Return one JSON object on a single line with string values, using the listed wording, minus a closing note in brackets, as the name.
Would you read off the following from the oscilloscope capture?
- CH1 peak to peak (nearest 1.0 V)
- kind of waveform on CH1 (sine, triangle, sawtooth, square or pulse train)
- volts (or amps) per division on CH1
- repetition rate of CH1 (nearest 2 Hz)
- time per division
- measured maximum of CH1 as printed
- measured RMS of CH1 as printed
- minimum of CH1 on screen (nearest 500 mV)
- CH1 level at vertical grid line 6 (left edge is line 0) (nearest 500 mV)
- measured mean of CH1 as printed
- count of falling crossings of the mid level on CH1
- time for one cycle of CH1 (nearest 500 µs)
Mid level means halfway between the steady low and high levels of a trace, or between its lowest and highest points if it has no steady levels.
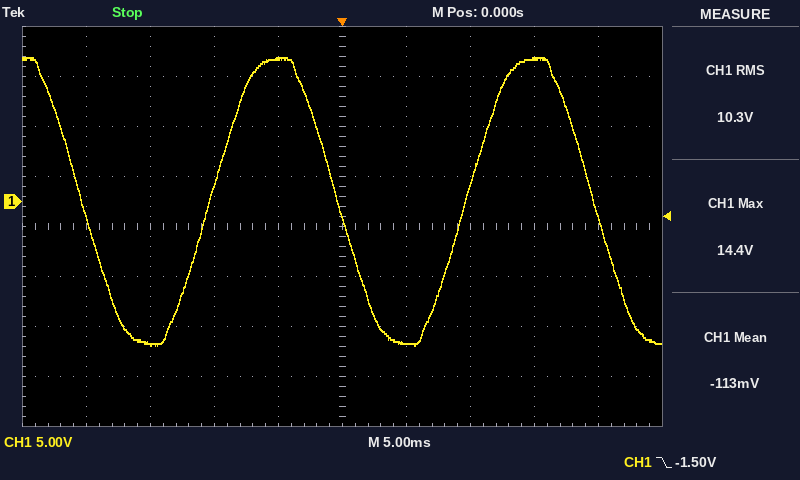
{"CH1 peak to peak": "29.0 V", "kind of waveform on CH1": "sine", "volts (or amps) per division on CH1": "5 V", "repetition rate of CH1": "50 Hz", "time per division": "5 ms", "measured maximum of CH1 as printed": "14.4 V", "measured RMS of CH1 as printed": "10.3 V", "minimum of CH1 on screen": "-14.5 V", "CH1 level at vertical grid line 6 (left edge is line 0)": "-14.0 V", "measured mean of CH1 as printed": "-113 mV", "count of falling crossings of the mid level on CH1": "3", "time for one cycle of CH1": "20.0 ms"}
